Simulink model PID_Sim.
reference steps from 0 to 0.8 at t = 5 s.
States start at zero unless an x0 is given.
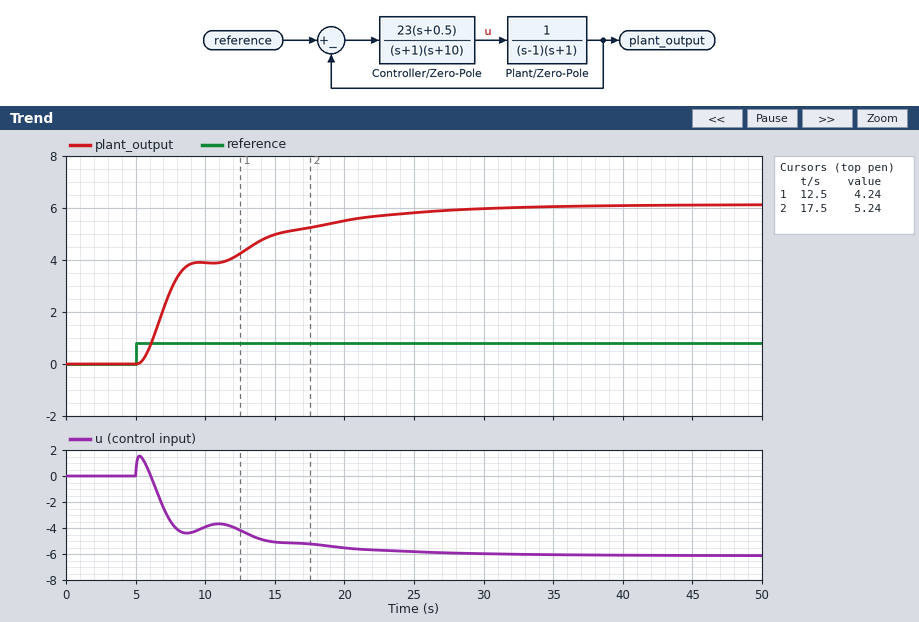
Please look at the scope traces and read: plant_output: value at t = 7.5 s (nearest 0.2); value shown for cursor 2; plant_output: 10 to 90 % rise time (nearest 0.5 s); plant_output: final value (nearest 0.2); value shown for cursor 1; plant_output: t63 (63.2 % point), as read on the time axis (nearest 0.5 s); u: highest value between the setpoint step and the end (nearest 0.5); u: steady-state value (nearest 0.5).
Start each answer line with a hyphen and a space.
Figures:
- 2.8
- 5.24
- 14.0 s
- 6.2
- 4.24
- 9.0 s
- 1.5
- -6.0
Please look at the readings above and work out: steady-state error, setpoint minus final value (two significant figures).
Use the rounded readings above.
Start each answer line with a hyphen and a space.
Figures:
- -5.4
